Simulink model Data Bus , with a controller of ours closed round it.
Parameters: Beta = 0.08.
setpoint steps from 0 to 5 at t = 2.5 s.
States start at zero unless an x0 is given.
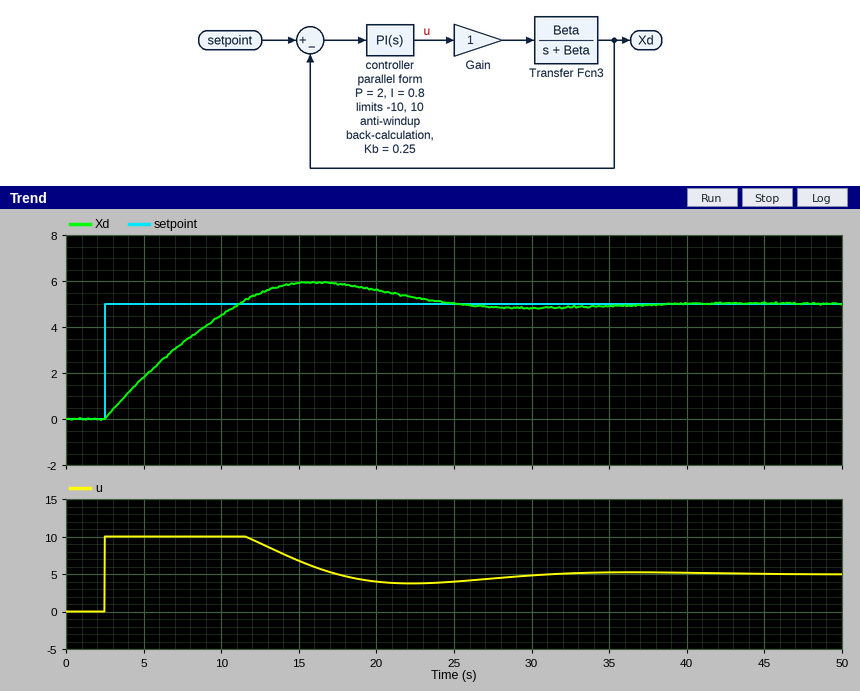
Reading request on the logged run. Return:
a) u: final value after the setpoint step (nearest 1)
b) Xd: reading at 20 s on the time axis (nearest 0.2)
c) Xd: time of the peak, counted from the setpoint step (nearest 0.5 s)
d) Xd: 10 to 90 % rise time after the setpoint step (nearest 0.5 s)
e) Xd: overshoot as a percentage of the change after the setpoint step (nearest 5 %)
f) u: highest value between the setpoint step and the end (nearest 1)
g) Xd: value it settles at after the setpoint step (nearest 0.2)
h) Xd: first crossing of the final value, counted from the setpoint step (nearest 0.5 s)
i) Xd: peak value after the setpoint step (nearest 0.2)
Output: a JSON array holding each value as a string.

["5", "5.6", "13.5 s", "7.0 s", "20 %", "10", "5.0", "8.5 s", "6.0"]
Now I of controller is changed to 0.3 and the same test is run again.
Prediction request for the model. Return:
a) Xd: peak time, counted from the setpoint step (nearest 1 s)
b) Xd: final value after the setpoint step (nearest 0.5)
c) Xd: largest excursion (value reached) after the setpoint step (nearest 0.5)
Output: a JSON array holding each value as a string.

["19 s", "5.0", "5.5"]
